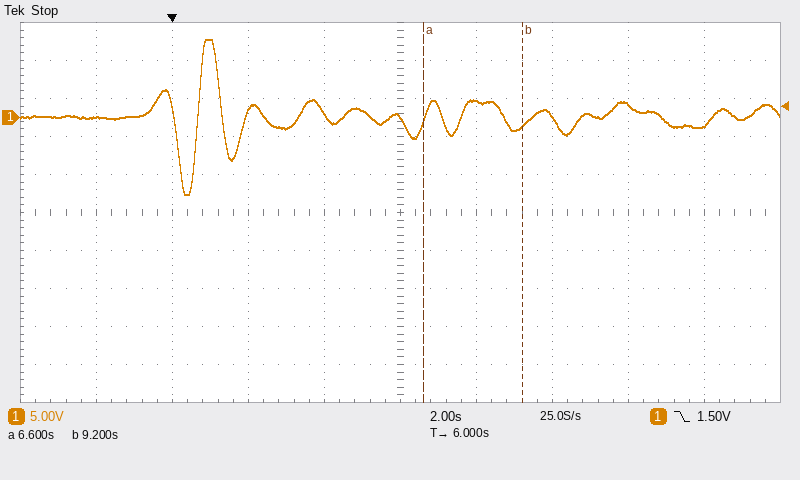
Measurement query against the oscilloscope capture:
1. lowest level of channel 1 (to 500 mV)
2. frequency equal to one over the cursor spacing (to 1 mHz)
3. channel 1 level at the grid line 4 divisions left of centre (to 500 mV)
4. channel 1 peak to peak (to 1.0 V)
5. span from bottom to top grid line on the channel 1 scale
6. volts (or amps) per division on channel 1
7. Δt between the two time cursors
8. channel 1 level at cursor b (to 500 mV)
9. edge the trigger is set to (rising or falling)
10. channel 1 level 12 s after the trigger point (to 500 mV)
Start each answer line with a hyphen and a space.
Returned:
- -10.0 V
- 385 mHz
- 0.0 V
- 20.0 V
- 50 V
- 5 V
- 2.6 s
- -1.0 V
- falling
- 1.5 V
